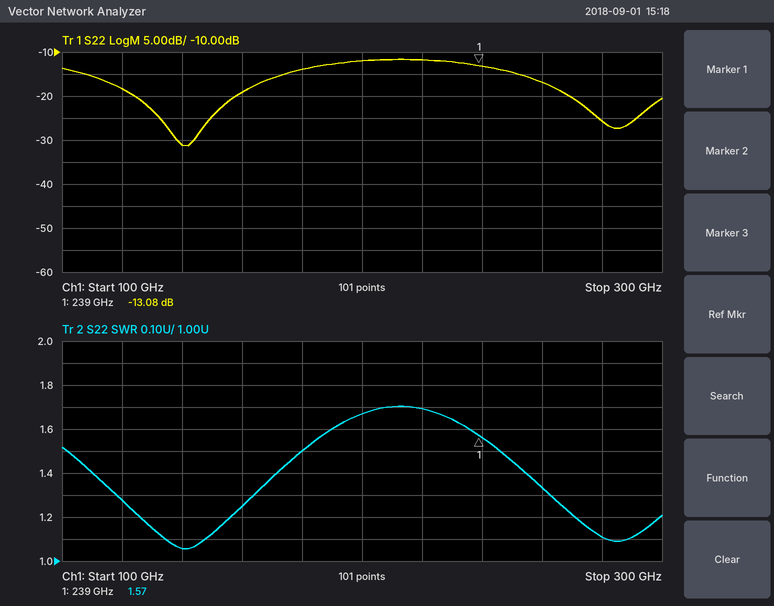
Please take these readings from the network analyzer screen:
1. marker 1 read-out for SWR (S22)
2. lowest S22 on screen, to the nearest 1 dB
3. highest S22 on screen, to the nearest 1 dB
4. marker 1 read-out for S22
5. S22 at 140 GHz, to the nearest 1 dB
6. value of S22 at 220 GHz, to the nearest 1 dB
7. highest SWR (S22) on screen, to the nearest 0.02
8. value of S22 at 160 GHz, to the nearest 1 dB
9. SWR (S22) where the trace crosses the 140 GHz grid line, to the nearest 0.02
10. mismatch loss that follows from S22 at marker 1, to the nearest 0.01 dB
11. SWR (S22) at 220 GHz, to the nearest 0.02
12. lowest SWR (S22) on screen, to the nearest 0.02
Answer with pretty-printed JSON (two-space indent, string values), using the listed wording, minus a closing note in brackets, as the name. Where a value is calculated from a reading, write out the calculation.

{
  "marker 1 read-out for SWR": "1.57",
  "lowest S22 on screen, to the nearest 1 dB": "-31 dB",
  "highest S22 on screen, to the nearest 1 dB": "-12 dB",
  "marker 1 read-out for S22": "-13.08 dB",
  "S22 at 140 GHz, to the nearest 1 dB": "-31 dB",
  "value of S22 at 220 GHz, to the nearest 1 dB": "-12 dB",
  "highest SWR (S22) on screen, to the nearest 0.02": "1.70",
  "value of S22 at 160 GHz, to the nearest 1 dB": "-19 dB",
  "SWR (S22) where the trace crosses the 140 GHz grid line, to the nearest 0.02": "1.06",
  "mismatch loss that follows from S22 at marker 1, to the nearest 0.01 dB": "−10 log10(1 − 10^(-13.08/10)) ≈ 0.22 dB",
  "SWR (S22) at 220 GHz, to the nearest 0.02": "1.70",
  "lowest SWR (S22) on screen, to the nearest 0.02": "1.06"
}
